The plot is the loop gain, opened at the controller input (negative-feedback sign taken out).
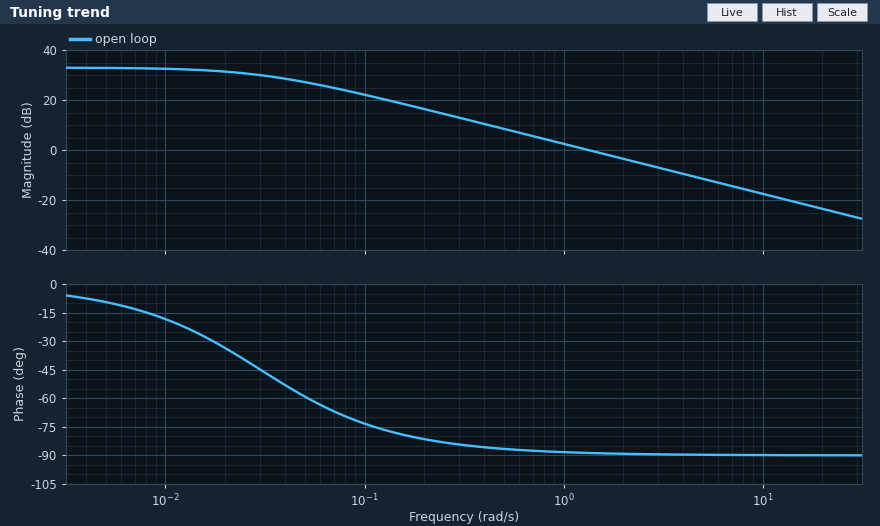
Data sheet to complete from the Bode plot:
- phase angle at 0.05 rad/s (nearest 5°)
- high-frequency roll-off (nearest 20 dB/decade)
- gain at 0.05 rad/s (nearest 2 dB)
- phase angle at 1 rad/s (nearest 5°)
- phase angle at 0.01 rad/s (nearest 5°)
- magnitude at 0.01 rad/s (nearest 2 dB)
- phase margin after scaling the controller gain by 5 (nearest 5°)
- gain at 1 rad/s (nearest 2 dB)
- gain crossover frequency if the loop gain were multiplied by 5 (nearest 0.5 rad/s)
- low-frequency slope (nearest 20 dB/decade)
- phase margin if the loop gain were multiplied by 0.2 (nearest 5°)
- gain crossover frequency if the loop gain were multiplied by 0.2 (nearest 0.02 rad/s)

-60°
-20 dB/decade
28 dB
-90°
-20°
32 dB
90°
2 dB
6.5 rad/s
0 dB/decade
95°
0.26 rad/s
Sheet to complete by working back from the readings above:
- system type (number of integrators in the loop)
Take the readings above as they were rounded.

0
